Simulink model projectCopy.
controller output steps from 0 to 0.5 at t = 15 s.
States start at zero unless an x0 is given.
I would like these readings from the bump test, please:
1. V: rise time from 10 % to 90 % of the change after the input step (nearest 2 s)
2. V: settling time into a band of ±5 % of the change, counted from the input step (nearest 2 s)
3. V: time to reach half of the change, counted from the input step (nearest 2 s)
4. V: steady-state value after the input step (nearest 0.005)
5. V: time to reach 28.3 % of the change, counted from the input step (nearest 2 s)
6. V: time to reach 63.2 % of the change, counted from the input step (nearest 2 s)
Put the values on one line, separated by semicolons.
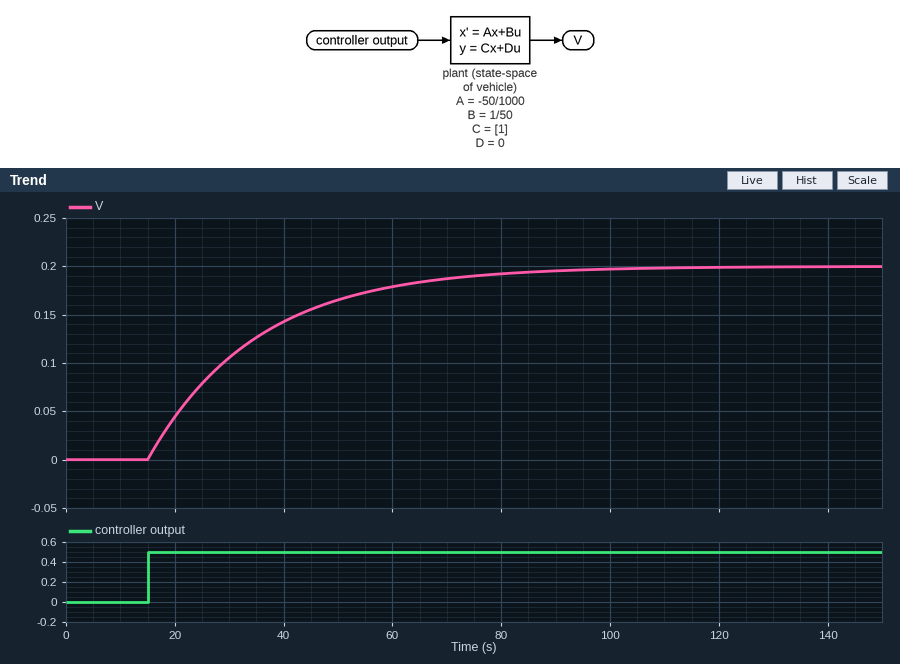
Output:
44 s; 60 s; 14 s; 0.200; 6 s; 20 s
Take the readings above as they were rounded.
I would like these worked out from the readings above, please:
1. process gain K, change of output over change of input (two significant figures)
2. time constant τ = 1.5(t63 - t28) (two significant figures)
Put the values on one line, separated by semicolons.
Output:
0.40; 21 s
